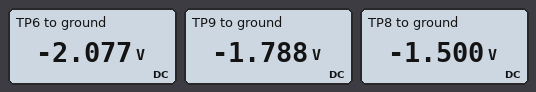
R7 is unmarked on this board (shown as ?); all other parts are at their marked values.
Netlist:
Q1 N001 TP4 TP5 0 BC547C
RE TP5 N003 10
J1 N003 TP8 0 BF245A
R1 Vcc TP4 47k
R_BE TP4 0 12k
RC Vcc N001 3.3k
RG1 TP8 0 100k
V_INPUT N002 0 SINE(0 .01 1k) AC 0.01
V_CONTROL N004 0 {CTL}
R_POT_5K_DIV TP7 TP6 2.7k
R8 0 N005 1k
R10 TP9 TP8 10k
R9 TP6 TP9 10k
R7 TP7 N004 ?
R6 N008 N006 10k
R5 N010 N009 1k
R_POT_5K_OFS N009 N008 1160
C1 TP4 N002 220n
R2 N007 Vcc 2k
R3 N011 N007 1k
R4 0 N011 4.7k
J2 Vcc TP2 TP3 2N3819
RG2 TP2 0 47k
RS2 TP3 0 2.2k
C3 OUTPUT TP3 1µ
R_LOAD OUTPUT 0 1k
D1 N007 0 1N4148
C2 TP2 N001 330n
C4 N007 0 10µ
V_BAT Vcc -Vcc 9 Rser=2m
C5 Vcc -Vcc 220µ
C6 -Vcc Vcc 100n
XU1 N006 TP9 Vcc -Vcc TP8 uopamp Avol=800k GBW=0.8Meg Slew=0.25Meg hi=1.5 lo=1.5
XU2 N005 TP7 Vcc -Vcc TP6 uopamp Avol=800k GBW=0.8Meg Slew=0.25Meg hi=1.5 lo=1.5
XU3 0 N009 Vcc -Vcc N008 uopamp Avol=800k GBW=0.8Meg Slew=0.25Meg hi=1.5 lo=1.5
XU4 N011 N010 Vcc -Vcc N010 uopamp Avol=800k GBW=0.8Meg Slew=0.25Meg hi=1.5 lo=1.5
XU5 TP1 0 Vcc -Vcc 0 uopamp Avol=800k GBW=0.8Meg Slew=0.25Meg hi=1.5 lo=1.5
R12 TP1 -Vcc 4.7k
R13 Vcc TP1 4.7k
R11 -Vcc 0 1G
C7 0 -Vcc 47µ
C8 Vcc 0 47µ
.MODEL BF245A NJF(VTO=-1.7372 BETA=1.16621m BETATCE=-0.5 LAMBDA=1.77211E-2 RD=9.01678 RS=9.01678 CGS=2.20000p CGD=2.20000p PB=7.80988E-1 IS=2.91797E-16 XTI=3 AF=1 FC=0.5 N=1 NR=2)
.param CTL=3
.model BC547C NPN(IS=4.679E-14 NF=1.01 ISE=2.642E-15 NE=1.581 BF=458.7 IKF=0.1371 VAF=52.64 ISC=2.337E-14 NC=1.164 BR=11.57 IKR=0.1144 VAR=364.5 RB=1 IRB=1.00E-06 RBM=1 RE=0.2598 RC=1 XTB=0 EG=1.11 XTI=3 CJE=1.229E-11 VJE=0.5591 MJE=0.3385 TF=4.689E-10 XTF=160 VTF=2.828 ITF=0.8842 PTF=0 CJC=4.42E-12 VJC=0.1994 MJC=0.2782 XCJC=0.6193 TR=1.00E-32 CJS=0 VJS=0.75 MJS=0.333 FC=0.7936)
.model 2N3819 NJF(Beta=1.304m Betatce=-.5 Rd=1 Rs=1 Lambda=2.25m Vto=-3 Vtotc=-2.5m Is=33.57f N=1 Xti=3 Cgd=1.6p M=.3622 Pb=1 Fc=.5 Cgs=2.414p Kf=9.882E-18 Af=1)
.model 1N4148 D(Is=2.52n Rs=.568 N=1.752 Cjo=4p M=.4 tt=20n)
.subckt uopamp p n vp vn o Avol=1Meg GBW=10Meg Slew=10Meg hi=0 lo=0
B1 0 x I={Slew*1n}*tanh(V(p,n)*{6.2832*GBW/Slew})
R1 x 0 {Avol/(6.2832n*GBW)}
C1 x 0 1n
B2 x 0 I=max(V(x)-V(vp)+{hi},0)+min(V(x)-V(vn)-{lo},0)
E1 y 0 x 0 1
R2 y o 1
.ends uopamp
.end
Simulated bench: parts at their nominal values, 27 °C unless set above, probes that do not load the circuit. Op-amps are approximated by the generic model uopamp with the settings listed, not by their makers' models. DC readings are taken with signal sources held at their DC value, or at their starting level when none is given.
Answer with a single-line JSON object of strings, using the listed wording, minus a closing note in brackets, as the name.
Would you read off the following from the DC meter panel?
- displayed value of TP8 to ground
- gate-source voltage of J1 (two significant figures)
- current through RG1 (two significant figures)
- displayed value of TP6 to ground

{"displayed value of TP8 to ground": "-1.500 V", "gate-source voltage of J1": "-1.5 V", "current through RG1": "15 µA", "displayed value of TP6 to ground": "-2.077 V"}
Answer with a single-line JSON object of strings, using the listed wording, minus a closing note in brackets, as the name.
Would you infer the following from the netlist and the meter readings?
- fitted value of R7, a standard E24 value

{"fitted value of R7, a standard E24 value": "3.9 kΩ"}
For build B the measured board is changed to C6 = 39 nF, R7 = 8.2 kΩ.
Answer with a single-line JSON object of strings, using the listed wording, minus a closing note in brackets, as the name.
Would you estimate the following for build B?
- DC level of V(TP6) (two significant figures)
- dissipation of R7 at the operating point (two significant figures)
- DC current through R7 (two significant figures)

{"DC level of V(TP6)": "-1.5 V", "dissipation of R7 at the operating point": "1.4 mW", "DC current through R7": "410 µA"}
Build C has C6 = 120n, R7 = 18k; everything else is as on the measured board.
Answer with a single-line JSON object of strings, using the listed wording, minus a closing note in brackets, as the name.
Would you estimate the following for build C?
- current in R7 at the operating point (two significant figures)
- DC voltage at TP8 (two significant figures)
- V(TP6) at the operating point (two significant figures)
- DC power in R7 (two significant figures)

{"current in R7 at the operating point": "220 µA", "DC voltage at TP8": "-1.5 V", "V(TP6) at the operating point": "-1.5 V", "DC power in R7": "850 µW"}
